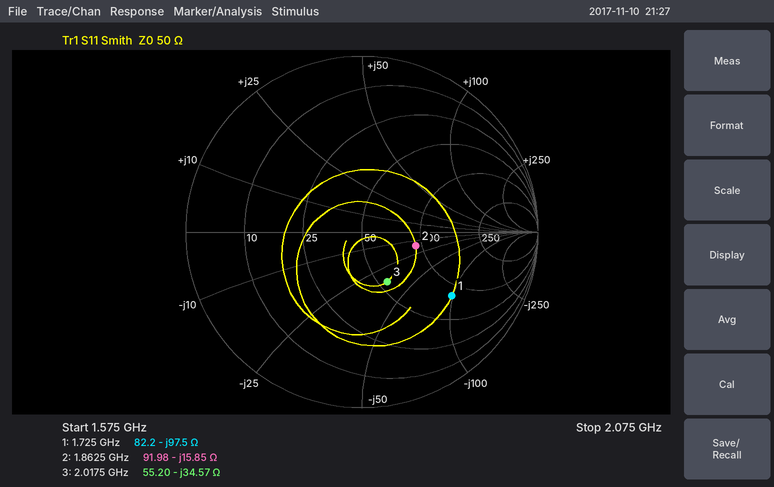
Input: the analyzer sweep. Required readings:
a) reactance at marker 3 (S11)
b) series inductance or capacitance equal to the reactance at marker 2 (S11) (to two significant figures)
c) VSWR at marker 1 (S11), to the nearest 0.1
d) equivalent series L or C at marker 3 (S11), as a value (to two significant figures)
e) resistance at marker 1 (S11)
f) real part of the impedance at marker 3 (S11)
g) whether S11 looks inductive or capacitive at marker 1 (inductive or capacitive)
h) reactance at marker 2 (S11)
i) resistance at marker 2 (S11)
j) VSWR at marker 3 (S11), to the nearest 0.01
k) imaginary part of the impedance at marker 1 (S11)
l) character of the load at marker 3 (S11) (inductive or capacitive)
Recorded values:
-34.57 Ω
5.4 pF
4.3
2.3 pF
82.2 Ω
55.20 Ω
capacitive
-15.85 Ω
91.98 Ω
1.92
-97.5 Ω
capacitive
